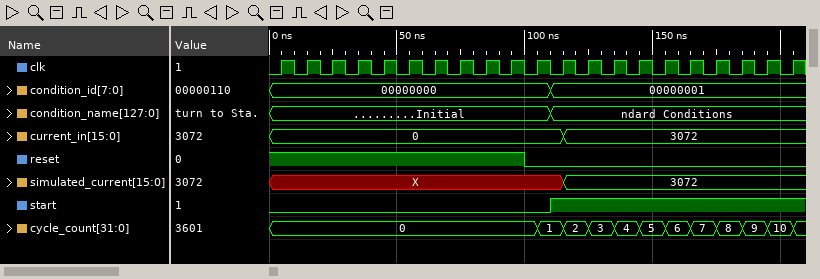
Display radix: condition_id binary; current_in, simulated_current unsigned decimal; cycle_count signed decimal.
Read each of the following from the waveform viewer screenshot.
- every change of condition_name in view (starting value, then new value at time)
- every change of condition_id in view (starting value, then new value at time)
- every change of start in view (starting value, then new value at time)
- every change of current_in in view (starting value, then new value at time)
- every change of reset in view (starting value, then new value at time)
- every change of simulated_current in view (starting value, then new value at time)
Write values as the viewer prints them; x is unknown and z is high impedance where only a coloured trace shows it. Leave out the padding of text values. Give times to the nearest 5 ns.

Initial, ndard Conditions at 110 ns
00000000, 00000001 at 110 ns
0, 1 at 110 ns
0, 3072 at 115 ns
1, 0 at 100 ns
X, 3072 at 115 ns
